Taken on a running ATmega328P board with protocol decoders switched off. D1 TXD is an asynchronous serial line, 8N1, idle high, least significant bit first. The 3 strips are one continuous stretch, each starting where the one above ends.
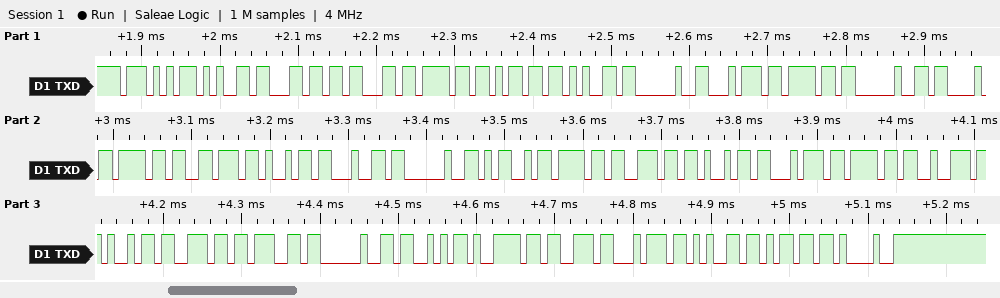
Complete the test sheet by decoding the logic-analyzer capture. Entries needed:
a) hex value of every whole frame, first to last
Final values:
57 65 6C 63 6F 6D 65 20 74 6F 20 43 6F 76 69 64 20 4D 6F 6E 69 74 6F 72 69 6E 67 20 53 79 73 74 65 6D 21
